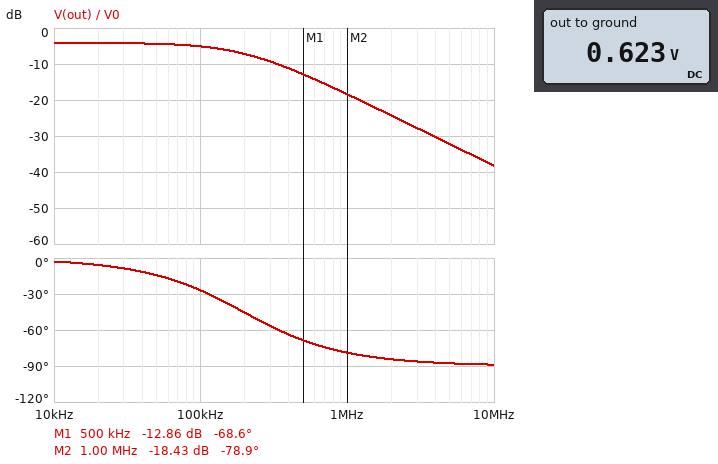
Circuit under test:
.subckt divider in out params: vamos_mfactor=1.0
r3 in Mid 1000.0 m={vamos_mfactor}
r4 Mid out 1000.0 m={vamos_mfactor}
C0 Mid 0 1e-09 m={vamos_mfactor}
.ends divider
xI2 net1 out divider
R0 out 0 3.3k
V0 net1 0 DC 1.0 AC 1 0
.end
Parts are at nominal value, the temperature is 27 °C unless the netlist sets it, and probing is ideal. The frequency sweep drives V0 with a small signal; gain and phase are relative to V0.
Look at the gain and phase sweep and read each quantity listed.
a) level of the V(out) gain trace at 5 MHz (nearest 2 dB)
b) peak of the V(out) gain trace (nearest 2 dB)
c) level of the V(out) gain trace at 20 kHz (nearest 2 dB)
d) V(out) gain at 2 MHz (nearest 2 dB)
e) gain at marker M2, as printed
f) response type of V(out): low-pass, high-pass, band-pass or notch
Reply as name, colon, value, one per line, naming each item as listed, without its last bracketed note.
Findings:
level of the V(out) gain trace at 5 MHz: -32 dB
peak of the V(out) gain trace: -4 dB
level of the V(out) gain trace at 20 kHz: -4 dB
V(out) gain at 2 MHz: -24 dB
gain at marker M2, as printed: -18.43 dB
response type of V(out): low-pass, high-pass, band-pass or notch: low-pass
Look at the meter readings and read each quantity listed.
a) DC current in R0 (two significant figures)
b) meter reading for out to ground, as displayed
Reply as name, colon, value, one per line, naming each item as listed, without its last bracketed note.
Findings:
DC current in R0: 190 µA
meter reading for out to ground, as displayed: 0.623 V
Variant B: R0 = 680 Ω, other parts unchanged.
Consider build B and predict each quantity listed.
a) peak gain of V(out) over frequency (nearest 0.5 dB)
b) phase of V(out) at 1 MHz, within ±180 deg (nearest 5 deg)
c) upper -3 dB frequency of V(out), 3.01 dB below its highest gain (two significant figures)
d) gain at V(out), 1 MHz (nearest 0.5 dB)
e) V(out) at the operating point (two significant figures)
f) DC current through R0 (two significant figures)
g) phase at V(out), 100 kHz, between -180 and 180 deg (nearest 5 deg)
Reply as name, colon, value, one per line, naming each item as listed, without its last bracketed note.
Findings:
peak gain of V(out) over frequency: -12.0 dB
phase of V(out) at 1 MHz, within ±180 deg: -75 deg
upper -3 dB frequency of V(out), 3.01 dB below its highest gain: 250 kHz
gain at V(out), 1 MHz: -24.0 dB
V(out) at the operating point: 250 mV
DC current through R0: 370 µA
phase at V(out), 100 kHz, between -180 and 180 deg: -20 deg
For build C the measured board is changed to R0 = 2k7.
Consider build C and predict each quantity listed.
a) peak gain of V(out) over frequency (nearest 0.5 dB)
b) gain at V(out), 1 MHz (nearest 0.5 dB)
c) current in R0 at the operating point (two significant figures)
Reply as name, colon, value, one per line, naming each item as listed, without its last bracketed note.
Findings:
peak gain of V(out) over frequency: -5.0 dB
gain at V(out), 1 MHz: -19.0 dB
current in R0 at the operating point: 210 µA
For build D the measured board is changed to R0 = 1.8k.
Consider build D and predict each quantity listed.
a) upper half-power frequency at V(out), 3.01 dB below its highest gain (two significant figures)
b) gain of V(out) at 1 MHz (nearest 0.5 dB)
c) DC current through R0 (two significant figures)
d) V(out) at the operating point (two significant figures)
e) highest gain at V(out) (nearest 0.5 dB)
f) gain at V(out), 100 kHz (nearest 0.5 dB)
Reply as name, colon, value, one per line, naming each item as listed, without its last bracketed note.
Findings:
upper half-power frequency at V(out), 3.01 dB below its highest gain: 220 kHz
gain of V(out) at 1 MHz: -20.0 dB
DC current through R0: 260 µA
V(out) at the operating point: 470 mV
highest gain at V(out): -6.5 dB
gain at V(out), 100 kHz: -7.5 dB
